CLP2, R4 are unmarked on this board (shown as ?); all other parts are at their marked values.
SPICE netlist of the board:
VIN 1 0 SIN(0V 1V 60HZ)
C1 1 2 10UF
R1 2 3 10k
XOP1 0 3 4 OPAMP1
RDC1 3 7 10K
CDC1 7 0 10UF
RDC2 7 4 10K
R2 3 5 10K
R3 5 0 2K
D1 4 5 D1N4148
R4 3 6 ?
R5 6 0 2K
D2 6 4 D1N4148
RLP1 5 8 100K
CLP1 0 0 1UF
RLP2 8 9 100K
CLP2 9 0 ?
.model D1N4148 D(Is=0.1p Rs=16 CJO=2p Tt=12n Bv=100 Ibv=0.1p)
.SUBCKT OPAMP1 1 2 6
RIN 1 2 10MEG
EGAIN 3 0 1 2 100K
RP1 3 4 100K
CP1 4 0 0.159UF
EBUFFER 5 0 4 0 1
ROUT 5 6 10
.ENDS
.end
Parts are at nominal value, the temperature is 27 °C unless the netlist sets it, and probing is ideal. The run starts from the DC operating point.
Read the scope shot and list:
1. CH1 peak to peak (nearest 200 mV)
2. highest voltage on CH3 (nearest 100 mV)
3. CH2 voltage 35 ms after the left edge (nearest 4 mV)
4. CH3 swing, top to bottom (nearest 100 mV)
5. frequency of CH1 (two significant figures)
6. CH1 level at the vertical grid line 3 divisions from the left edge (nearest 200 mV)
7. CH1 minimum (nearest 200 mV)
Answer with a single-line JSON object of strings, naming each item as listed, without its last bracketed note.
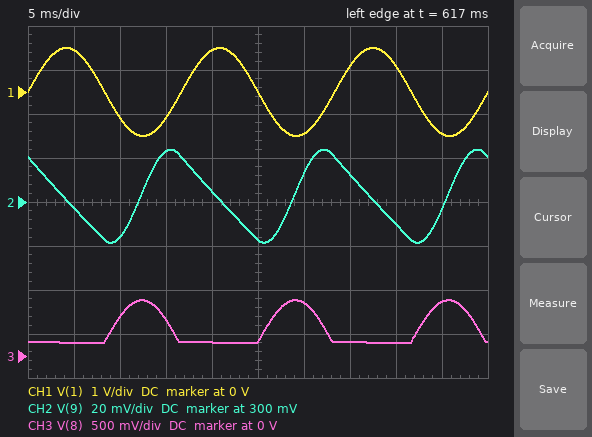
{"CH1 peak to peak": "2.0 V", "highest voltage on CH3": "600 mV", "CH2 voltage 35 ms after the left edge": "312 mV", "CH3 swing, top to bottom": "500 mV", "frequency of CH1": "60 Hz", "CH1 level at the vertical grid line 3 divisions from the left edge": "-600 mV", "CH1 minimum": "-1.0 V"}
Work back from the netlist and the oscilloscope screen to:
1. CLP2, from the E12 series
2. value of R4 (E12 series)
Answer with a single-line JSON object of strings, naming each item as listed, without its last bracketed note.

{"CLP2, from the E12 series": "330 nF", "value of R4": "6.8 kΩ"}
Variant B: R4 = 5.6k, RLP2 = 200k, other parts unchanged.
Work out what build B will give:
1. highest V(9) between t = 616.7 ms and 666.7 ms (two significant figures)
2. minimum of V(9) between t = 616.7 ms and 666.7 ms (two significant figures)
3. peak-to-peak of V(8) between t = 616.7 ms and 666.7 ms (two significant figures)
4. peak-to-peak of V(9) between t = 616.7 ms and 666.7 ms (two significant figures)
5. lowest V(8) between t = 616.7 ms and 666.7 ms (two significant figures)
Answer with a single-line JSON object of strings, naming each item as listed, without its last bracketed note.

{"highest V(9) between t = 616.7 ms and 666.7 ms": "310 mV", "minimum of V(9) between t = 616.7 ms and 666.7 ms": "280 mV", "peak-to-peak of V(8) between t = 616.7 ms and 666.7 ms": "640 mV", "peak-to-peak of V(9) between t = 616.7 ms and 666.7 ms": "28 mV", "lowest V(8) between t = 616.7 ms and 666.7 ms": "95 mV"}
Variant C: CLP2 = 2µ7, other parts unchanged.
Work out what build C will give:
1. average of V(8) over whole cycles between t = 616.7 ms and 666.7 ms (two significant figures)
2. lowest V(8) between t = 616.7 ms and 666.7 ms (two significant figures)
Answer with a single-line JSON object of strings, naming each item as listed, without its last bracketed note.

{"average of V(8) over whole cycles between t = 616.7 ms and 666.7 ms": "260 mV", "lowest V(8) between t = 616.7 ms and 666.7 ms": "100 mV"}
